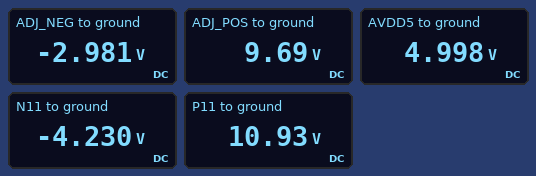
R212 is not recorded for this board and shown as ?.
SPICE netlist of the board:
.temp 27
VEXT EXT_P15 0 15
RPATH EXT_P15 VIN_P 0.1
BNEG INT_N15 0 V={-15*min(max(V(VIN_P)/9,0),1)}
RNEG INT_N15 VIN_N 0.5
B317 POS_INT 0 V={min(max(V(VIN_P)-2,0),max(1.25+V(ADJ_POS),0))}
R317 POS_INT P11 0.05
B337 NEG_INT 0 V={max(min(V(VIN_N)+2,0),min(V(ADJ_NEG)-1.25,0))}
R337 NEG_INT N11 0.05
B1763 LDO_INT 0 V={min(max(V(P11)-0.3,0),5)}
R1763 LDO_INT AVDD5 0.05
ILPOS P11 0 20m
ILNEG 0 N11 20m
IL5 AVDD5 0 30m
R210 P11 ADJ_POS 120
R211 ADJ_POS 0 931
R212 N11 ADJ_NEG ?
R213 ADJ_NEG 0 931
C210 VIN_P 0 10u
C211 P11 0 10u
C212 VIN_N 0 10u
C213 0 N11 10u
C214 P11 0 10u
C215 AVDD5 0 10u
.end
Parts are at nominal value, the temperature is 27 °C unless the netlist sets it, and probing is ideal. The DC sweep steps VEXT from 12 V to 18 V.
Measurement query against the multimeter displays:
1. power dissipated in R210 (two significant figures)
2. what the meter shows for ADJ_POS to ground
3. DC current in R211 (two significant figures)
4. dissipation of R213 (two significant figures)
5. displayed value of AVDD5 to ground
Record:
13 mW
9.69 V
10 mA
9.5 mW
4.998 V
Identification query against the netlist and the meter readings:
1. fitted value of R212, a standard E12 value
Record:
390 Ω
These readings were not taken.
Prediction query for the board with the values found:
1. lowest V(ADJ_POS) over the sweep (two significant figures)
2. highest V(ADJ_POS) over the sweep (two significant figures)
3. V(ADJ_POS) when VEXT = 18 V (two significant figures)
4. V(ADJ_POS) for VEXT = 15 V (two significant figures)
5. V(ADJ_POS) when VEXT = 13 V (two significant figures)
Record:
8.9 V
9.7 V
9.7 V
9.7 V
9.7 V
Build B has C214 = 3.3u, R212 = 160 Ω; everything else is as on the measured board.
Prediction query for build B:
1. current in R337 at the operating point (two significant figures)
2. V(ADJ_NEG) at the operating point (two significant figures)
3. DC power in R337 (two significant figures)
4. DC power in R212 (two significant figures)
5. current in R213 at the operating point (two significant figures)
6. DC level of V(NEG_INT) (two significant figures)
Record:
28 mA
-7.3 V
39 µW
9.7 mW
7.8 mA
-8.5 V
